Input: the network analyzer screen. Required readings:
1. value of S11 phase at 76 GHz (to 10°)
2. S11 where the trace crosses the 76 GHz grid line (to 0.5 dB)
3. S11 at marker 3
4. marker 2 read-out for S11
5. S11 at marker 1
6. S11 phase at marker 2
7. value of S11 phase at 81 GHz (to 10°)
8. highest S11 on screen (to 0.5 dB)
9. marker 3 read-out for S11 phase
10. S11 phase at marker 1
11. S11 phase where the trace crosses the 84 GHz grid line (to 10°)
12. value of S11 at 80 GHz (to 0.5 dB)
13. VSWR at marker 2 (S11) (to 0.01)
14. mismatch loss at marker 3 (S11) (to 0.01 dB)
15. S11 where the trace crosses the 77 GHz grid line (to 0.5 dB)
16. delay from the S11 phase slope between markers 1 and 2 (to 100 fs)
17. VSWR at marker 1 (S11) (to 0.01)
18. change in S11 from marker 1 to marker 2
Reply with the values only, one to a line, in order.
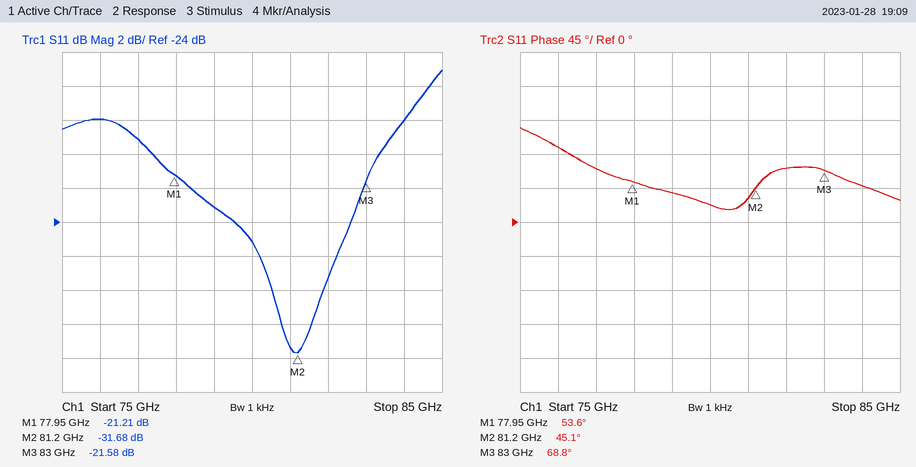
100°
-18.0 dB
-21.58 dB
-31.68 dB
-21.21 dB
45.1°
30°
-15.0 dB
68.8°
53.6°
50°
-25.0 dB
1.05
0.03 dB
-19.0 dB
7.3 ps
1.19
-10.47 dB
